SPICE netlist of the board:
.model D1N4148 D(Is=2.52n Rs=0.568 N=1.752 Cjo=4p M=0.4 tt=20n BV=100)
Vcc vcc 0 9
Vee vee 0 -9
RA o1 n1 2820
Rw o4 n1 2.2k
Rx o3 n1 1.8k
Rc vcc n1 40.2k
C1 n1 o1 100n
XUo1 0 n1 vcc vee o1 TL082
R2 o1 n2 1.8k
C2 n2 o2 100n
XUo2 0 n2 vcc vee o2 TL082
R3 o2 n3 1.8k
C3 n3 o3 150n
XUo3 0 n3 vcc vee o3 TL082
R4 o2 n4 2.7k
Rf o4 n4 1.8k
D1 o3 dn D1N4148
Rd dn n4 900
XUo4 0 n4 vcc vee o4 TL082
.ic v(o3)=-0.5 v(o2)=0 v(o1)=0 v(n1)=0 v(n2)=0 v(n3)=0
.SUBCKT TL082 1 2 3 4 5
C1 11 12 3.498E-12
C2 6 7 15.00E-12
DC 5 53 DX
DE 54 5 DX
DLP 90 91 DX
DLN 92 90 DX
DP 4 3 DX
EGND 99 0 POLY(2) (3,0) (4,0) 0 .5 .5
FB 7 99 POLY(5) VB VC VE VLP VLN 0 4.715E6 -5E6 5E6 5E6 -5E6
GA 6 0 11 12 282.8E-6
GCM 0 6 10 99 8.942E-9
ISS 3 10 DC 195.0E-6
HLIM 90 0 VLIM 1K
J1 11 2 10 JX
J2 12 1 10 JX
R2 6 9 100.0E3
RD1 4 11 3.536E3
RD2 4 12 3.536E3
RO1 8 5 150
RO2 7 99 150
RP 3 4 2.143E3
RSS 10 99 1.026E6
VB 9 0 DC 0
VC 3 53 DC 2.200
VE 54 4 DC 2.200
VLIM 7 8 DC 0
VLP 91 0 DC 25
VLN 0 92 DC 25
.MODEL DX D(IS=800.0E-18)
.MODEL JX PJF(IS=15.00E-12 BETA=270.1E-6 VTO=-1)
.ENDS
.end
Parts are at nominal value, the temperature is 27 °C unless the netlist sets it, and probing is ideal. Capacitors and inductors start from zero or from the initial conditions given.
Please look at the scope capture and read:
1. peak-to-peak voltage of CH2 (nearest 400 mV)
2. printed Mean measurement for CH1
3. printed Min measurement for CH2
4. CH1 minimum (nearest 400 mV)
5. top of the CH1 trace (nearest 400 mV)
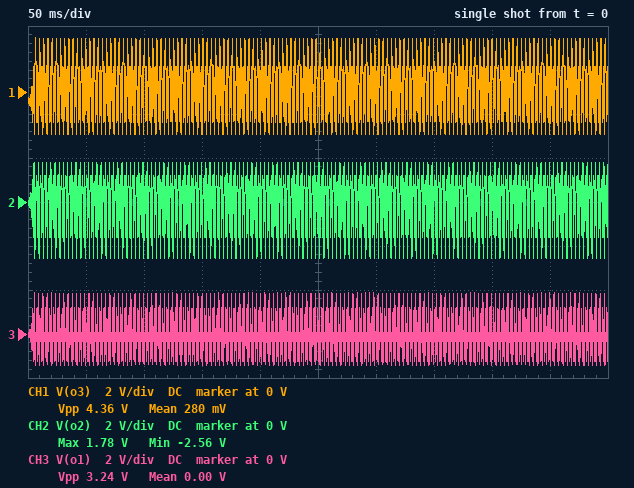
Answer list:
4.4 V
280 mV
-2.56 V
-2.0 V
2.4 V
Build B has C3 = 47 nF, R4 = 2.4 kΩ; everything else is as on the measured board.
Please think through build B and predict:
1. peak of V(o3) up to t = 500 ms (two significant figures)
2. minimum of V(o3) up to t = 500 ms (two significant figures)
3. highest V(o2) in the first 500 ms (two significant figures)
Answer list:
7.5 V
-7.4 V
3.5 V
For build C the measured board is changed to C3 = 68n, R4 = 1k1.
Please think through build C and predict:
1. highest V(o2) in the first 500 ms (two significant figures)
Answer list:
1.1 V
